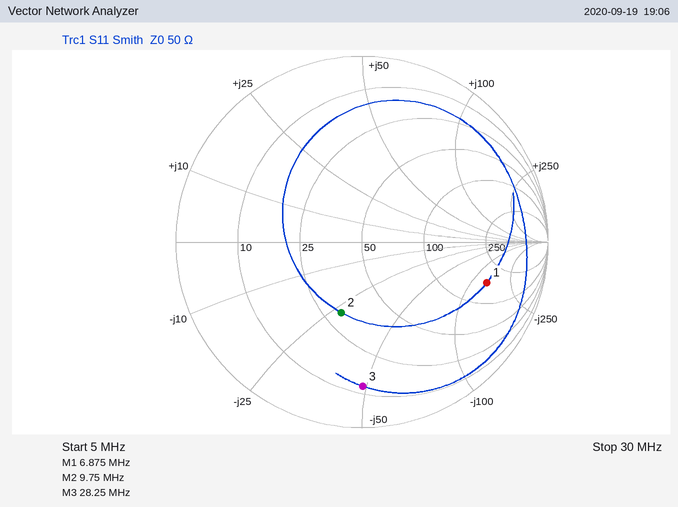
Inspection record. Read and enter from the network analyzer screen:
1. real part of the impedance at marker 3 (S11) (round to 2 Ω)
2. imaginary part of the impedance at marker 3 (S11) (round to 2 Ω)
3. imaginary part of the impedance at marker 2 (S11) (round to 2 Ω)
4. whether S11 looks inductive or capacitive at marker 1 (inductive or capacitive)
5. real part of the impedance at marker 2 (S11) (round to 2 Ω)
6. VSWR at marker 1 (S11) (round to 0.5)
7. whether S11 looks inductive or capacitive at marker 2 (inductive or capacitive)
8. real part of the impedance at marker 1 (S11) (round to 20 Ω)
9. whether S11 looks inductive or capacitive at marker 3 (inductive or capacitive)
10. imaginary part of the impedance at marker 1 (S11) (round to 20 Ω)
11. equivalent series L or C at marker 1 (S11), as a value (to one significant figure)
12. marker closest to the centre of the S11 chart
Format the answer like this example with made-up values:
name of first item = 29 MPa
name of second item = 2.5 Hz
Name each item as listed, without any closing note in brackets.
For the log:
real part of the impedance at marker 3 (S11) = 12 Ω
imaginary part of the impedance at marker 3 (S11) = -48 Ω
imaginary part of the impedance at marker 2 (S11) = -28 Ω
whether S11 looks inductive or capacitive at marker 1 = capacitive
real part of the impedance at marker 2 (S11) = 30 Ω
VSWR at marker 1 (S11) = 6.0
whether S11 looks inductive or capacitive at marker 2 = capacitive
real part of the impedance at marker 1 (S11) = 160 Ω
whether S11 looks inductive or capacitive at marker 3 = capacitive
imaginary part of the impedance at marker 1 (S11) = -140 Ω
equivalent series L or C at marker 1 (S11), as a value = 200 pF
marker closest to the centre of the S11 chart = marker 2
